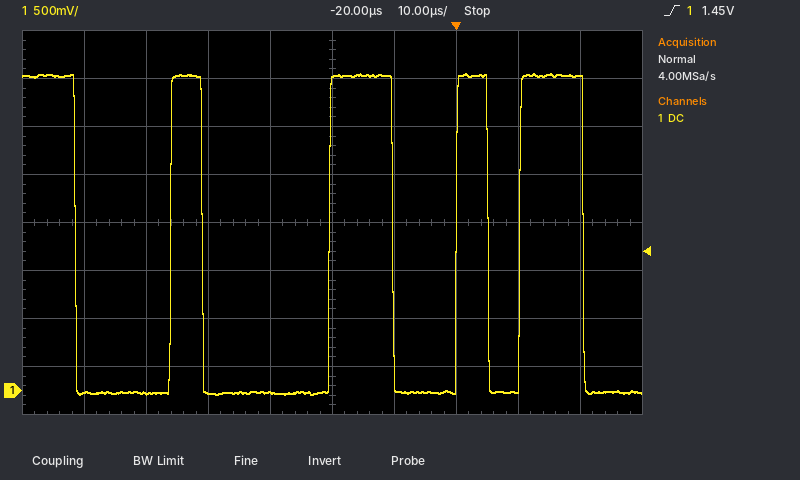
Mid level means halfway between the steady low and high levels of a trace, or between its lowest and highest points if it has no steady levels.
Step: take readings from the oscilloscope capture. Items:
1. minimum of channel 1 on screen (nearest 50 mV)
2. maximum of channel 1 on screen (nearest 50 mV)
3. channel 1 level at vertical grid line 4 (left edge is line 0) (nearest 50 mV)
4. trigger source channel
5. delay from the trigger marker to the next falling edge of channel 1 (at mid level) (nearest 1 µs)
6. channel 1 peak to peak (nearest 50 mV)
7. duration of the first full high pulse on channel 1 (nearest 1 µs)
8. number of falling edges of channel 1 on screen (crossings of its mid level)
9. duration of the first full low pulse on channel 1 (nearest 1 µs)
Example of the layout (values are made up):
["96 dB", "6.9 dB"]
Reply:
["-50 mV", "3.30 V", "0 mV", "channel 1", "5 µs", "3.35 V", "5 µs", "5", "15 µs"]
